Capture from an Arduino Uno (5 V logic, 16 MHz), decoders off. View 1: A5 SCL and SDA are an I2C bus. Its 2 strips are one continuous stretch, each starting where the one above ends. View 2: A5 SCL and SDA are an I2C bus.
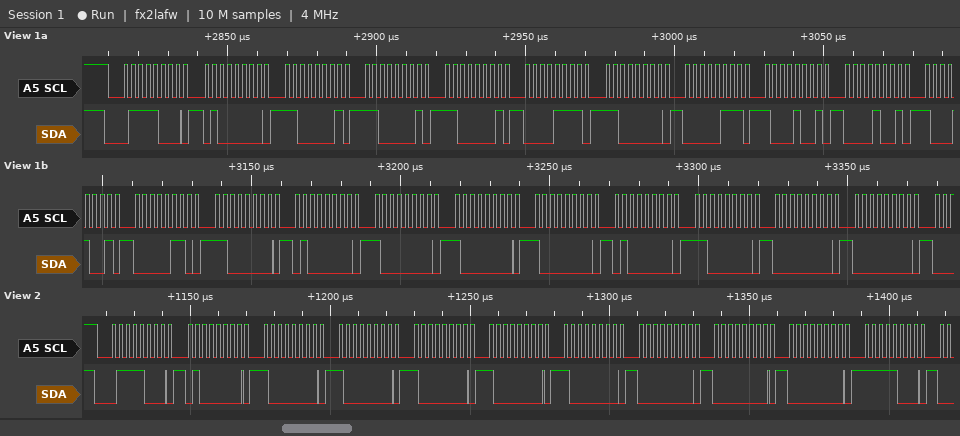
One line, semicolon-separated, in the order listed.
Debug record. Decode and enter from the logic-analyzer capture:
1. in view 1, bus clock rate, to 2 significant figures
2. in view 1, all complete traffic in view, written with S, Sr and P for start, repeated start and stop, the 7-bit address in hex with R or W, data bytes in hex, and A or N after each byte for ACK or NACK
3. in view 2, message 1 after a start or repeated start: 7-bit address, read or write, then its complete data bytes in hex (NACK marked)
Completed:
400 kHz; S 3CW A 40 A C1 A C1 A C1 A 0F A C0 A 07 A 89 A 09 A 89 A 06 A C0 A 40 A 80 A 80 A 80 A 40 A C0 A 00 A 00 A; 0x3C write: 40 80 80 80 80 80 00 00 00 F8
